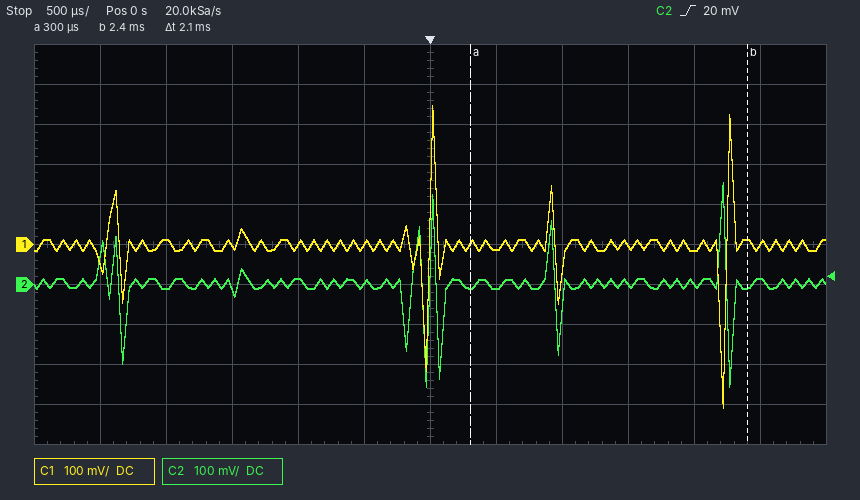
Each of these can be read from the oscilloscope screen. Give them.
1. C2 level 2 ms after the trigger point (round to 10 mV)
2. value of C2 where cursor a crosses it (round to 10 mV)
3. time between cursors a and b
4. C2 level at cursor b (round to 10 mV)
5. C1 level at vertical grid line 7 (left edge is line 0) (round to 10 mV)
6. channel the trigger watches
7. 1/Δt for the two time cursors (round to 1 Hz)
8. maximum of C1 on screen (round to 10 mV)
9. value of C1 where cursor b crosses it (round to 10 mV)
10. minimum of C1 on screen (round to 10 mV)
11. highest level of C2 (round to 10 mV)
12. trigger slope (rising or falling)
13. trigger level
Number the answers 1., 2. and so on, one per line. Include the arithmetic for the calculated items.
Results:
1. 0 mV
2. -10 mV
3. 2.1 ms
4. -10 mV
5. -10 mV
6. C2
7. 1 / 2.1 ms ≈ 476 Hz
8. 350 mV
9. 10 mV
10. -410 mV
11. 260 mV
12. rising
13. 20 mV
